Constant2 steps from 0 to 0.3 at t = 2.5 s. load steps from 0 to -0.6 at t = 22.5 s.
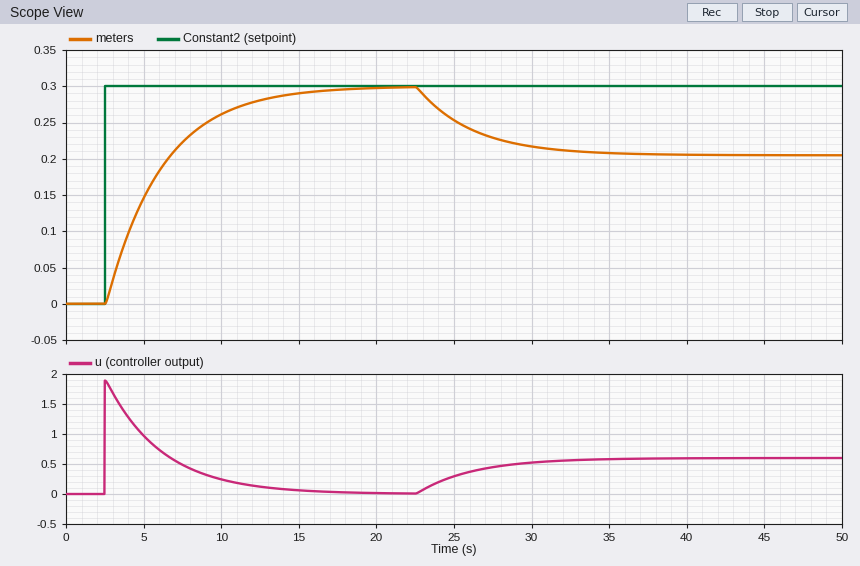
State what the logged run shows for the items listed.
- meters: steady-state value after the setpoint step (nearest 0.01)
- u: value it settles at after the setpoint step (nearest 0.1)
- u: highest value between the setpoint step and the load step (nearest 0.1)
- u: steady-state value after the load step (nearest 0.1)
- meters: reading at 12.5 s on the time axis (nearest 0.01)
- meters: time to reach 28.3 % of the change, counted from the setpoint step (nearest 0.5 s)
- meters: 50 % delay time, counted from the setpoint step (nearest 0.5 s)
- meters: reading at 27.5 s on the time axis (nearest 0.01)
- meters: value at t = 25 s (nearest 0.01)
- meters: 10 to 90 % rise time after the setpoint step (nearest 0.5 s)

0.30
0.0
1.9
0.6
0.28
1.5 s
2.5 s
0.23
0.25
8.0 s
